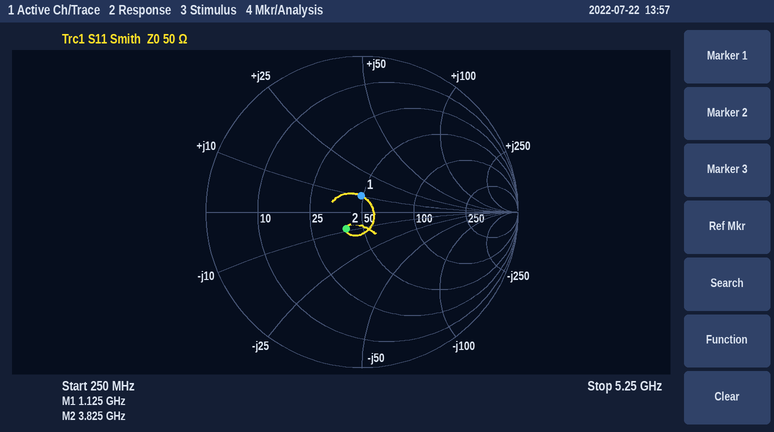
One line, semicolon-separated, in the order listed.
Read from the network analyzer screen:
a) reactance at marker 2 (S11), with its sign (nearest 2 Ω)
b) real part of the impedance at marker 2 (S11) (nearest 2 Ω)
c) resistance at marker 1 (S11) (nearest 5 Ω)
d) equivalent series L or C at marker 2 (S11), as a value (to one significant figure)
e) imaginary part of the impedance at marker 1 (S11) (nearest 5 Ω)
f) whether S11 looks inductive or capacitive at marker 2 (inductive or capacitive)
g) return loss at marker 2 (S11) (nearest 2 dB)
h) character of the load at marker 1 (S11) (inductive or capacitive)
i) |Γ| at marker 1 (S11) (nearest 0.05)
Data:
-8 Ω; 40 Ω; 50 Ω; 5 pF; +10 Ω; capacitive; 16 dB; inductive; 0.10
